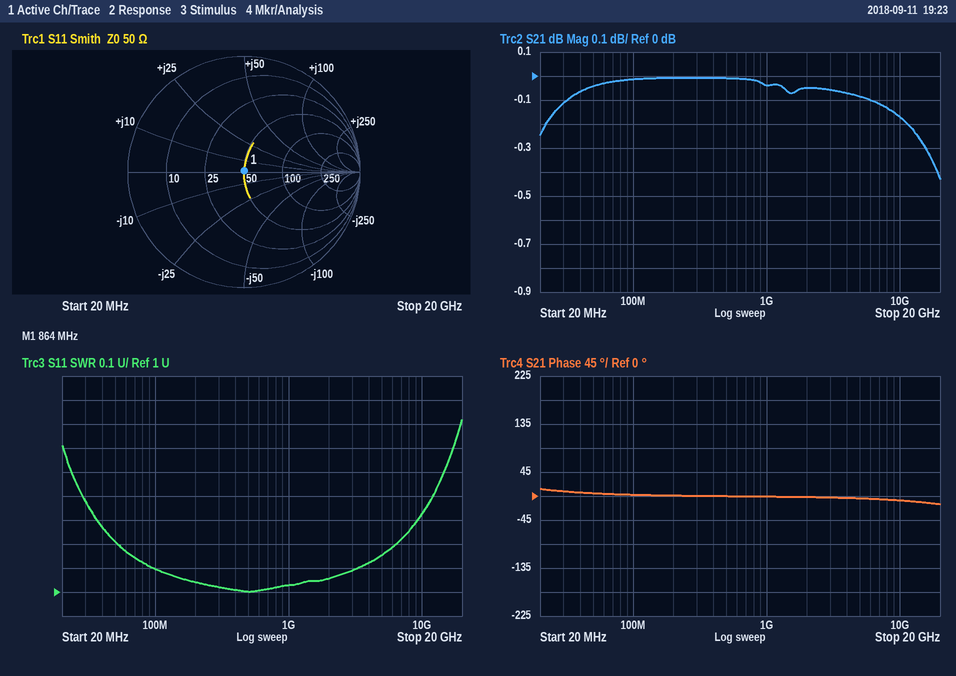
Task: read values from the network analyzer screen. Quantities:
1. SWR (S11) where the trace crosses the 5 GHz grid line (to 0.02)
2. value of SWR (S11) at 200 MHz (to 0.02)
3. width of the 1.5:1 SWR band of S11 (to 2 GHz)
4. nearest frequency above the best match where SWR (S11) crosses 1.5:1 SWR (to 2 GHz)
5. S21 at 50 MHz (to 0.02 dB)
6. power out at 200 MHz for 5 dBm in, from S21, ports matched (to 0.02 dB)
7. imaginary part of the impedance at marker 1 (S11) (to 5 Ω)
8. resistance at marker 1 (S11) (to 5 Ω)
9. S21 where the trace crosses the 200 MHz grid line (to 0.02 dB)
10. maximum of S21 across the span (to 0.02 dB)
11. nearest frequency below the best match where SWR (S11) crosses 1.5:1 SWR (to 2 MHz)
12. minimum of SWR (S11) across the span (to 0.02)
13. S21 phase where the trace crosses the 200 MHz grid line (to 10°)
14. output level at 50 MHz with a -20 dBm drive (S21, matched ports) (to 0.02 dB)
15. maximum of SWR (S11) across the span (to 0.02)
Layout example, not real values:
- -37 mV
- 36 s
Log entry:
- 1.16
- 1.04
- 14 GHz
- 14 GHz
- -0.04 dB
- 5.00 dBm
- 0 Ω
- 50 Ω
- 0.00 dB
- 0.00 dB
- 24 MHz
- 1.00
- 0°
- -20.04 dBm
- 1.72
